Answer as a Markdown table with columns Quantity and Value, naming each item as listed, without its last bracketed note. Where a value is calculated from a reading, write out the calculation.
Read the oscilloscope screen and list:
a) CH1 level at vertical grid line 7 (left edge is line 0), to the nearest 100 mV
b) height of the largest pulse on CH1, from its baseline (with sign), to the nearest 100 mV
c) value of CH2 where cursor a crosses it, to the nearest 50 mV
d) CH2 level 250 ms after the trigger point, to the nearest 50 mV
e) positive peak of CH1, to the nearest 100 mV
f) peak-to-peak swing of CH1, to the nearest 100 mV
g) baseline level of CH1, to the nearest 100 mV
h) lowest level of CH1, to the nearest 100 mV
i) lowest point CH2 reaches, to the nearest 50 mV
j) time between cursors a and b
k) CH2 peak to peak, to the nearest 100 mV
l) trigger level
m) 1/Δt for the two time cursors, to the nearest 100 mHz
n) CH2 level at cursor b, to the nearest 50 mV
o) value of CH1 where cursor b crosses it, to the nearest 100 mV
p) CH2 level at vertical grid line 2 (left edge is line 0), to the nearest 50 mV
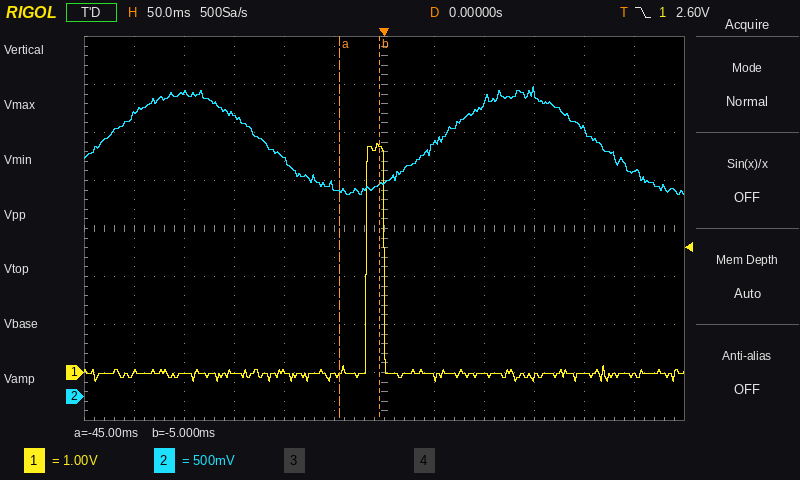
| Quantity | Value |
|---|---|
| CH1 level at vertical grid line 7 (left edge is line 0), to the nearest 100 mV | -100 mV |
| height of the largest pulse on CH1, from its baseline (with sign), to the nearest 100 mV | 4.8 V − (0.0 V) = +4.8 V |
| value of CH2 where cursor a crosses it, to the nearest 50 mV | 2.15 V |
| CH2 level 250 ms after the trigger point, to the nearest 50 mV | 2.35 V |
| positive peak of CH1, to the nearest 100 mV | 4.8 V |
| peak-to-peak swing of CH1, to the nearest 100 mV | 4.8 V − (-200 mV) = 5.0 V |
| baseline level of CH1, to the nearest 100 mV | 0.0 V |
| lowest level of CH1, to the nearest 100 mV | -200 mV |
| lowest point CH2 reaches, to the nearest 50 mV | 2.10 V |
| time between cursors a and b | -5 ms − (-45 ms) = 40 ms |
| CH2 peak to peak, to the nearest 100 mV | 1.10 V |
| trigger level | 2.60 V |
| 1/Δt for the two time cursors, to the nearest 100 mHz | 1 / 40 ms ≈ 25.0 Hz |
| CH2 level at cursor b, to the nearest 50 mV | 2.20 V |
| value of CH1 where cursor b crosses it, to the nearest 100 mV | 4.7 V |
| CH2 level at vertical grid line 2 (left edge is line 0), to the nearest 50 mV | 3.15 V |
